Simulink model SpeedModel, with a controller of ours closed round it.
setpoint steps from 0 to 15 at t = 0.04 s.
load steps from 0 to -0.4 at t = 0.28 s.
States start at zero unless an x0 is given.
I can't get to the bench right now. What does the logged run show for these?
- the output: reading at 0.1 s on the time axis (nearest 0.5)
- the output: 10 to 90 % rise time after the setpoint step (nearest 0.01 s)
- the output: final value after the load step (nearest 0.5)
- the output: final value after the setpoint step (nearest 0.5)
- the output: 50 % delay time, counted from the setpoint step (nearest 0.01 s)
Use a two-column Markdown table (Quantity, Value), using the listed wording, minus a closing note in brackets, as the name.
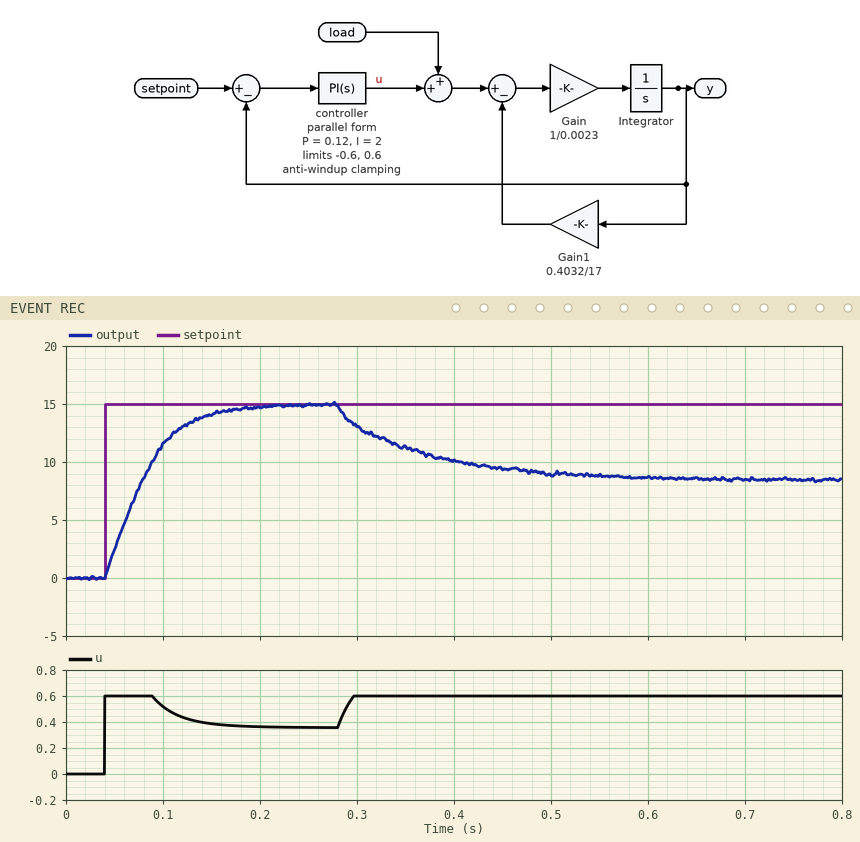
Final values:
| Quantity | Value |
|---|---|
| the output: reading at 0.1 s on the time axis | 11.5 |
| the output: 10 to 90 % rise time after the setpoint step | 0.08 s |
| the output: final value after the load step | 8.5 |
| the output: final value after the setpoint step | 15.0 |
| the output: 50 % delay time, counted from the setpoint step | 0.03 s |
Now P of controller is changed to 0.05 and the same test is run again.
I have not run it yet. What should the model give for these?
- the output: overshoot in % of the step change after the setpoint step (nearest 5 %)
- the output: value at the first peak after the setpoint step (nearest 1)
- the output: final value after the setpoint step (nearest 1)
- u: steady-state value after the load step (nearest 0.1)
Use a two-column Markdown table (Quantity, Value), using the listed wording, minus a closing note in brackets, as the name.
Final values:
| Quantity | Value |
|---|---|
| the output: overshoot in % of the step change after the setpoint step | 10 % |
| the output: value at the first peak after the setpoint step | 16 |
| the output: final value after the setpoint step | 15 |
| u: steady-state value after the load step | 0.6 |
